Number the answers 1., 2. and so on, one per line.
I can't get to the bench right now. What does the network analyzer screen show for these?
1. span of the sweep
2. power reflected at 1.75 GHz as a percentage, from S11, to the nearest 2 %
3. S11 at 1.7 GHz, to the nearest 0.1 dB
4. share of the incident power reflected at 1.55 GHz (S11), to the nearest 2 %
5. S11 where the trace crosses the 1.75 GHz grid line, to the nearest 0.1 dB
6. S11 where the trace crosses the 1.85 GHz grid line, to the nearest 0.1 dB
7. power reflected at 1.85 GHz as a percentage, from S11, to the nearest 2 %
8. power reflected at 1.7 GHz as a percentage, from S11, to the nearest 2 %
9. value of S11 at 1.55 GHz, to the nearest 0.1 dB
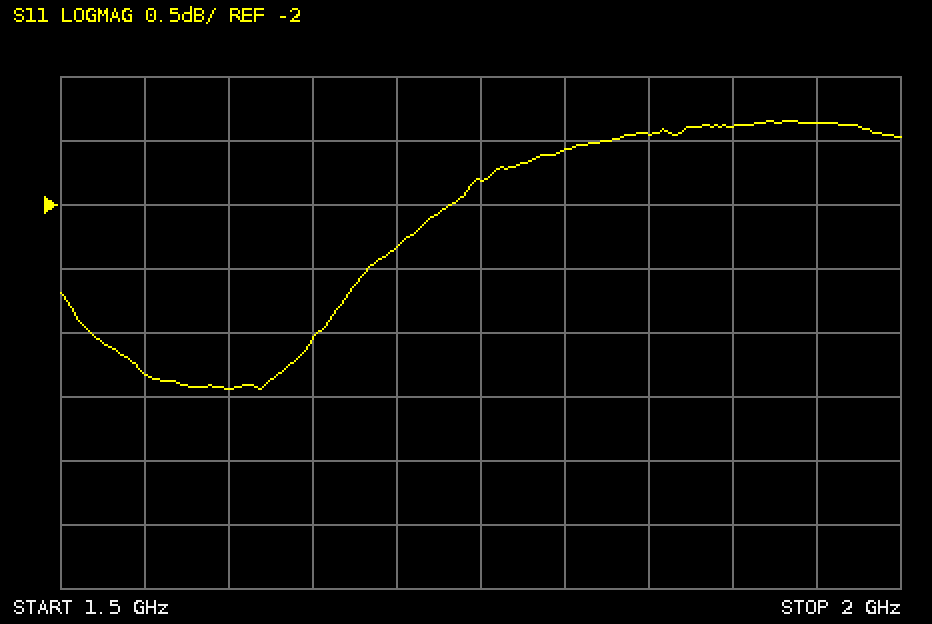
1. 500 MHz
2. 66 %
3. -2.3 dB
4. 46 %
5. -1.8 dB
6. -1.4 dB
7. 72 %
8. 58 %
9. -3.3 dB
